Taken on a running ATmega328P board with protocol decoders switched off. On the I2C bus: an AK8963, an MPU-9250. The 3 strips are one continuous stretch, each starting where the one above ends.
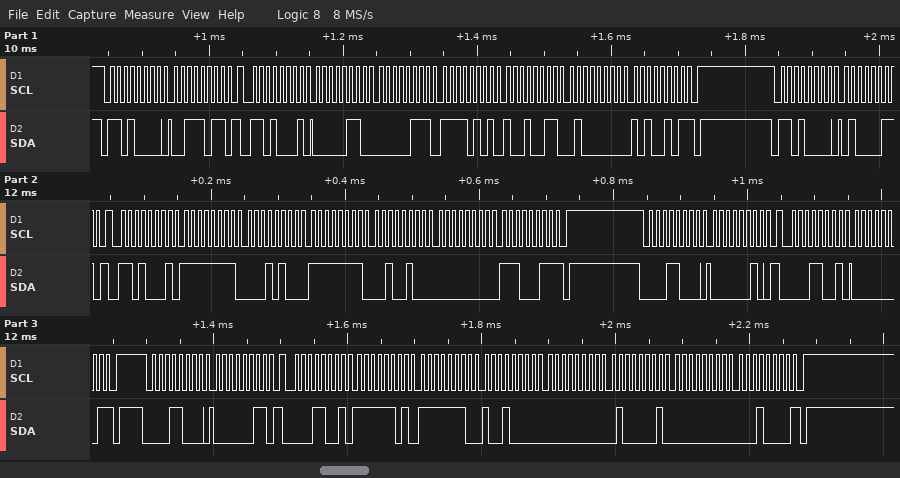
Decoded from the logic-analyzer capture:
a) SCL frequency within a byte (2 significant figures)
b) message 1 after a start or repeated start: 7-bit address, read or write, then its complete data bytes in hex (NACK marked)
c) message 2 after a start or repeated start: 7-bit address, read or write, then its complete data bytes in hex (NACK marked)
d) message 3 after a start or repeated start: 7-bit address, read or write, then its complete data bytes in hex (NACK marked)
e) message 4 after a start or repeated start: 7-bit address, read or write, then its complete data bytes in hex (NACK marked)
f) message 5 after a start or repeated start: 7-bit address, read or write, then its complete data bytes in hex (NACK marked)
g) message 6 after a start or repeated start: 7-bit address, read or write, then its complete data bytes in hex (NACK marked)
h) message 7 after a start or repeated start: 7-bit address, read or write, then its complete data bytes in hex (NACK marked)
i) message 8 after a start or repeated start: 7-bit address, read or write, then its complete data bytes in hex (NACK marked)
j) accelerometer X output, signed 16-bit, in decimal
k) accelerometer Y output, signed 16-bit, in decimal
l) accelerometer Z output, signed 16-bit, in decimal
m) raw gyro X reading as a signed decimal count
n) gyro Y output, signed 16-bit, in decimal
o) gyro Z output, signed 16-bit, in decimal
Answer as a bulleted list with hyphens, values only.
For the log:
- 100 kHz
- 0x68 write: 3B
- 0x68 read: 06 07 F5 93 40 A5 NACK
- 0x68 write: 43
- 0x68 read: FF 14 FF 24 00 E3 NACK
- 0x0C write: 02
- 0x0C read: 01 NACK
- 0x0C write: 03
- 0x0C read: FD FE 90 00 41 00 10 NACK
- 1543
- -2669
- 16549
- -236
- -220
- 227
